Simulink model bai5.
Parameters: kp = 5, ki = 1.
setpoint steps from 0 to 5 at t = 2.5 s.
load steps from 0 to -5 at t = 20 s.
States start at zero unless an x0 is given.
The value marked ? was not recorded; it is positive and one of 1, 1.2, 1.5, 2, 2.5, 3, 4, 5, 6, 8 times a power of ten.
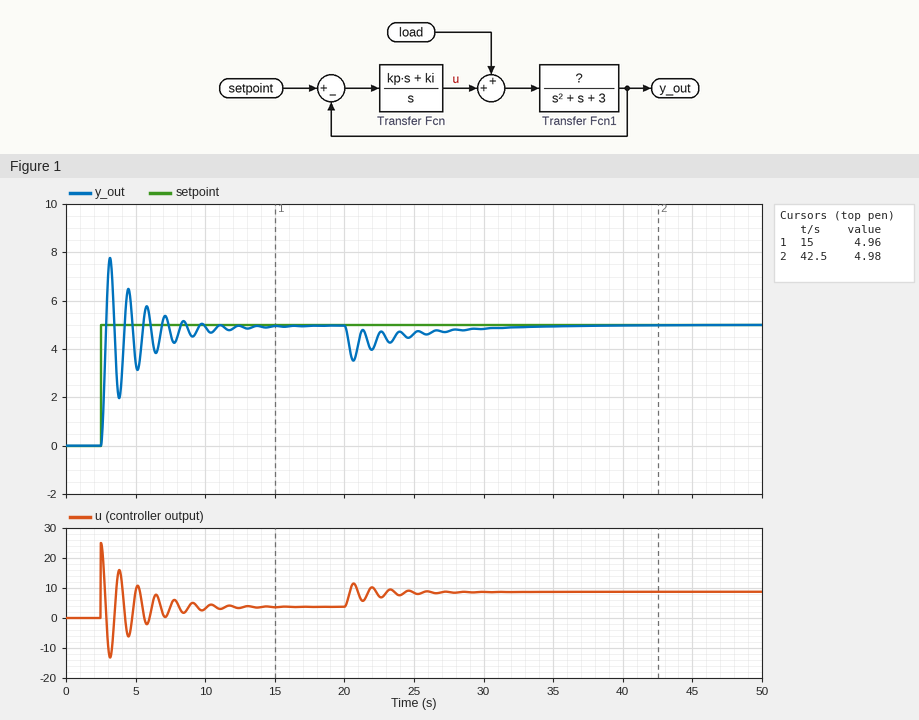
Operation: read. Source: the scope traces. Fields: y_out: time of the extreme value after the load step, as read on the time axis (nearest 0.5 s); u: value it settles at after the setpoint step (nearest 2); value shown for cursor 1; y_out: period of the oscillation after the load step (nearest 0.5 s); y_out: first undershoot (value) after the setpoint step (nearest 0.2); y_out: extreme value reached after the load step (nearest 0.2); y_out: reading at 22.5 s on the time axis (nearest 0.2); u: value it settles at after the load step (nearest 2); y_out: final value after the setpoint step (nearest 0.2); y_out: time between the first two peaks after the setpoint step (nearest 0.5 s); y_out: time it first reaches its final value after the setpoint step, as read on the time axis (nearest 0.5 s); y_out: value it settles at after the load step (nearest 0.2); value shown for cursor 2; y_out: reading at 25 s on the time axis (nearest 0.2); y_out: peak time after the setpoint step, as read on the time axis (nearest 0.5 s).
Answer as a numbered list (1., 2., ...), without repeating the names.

1. 20.5 s
2. 4
3. 4.96
4. 1.5 s
5. 2.0
6. 3.6
7. 4.6
8. 8
9. 5.0
10. 1.5 s
11. 3.0 s
12. 5.0
13. 4.98
14. 4.6
15. 3.0 s
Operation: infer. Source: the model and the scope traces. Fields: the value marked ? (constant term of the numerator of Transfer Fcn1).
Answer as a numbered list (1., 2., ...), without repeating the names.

1. 4
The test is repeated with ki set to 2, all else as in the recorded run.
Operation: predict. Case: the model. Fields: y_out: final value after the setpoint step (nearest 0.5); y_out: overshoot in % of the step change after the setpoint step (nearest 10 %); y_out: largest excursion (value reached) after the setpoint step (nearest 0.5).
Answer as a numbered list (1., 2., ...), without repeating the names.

1. 5.0
2. 60 %
3. 8.0
